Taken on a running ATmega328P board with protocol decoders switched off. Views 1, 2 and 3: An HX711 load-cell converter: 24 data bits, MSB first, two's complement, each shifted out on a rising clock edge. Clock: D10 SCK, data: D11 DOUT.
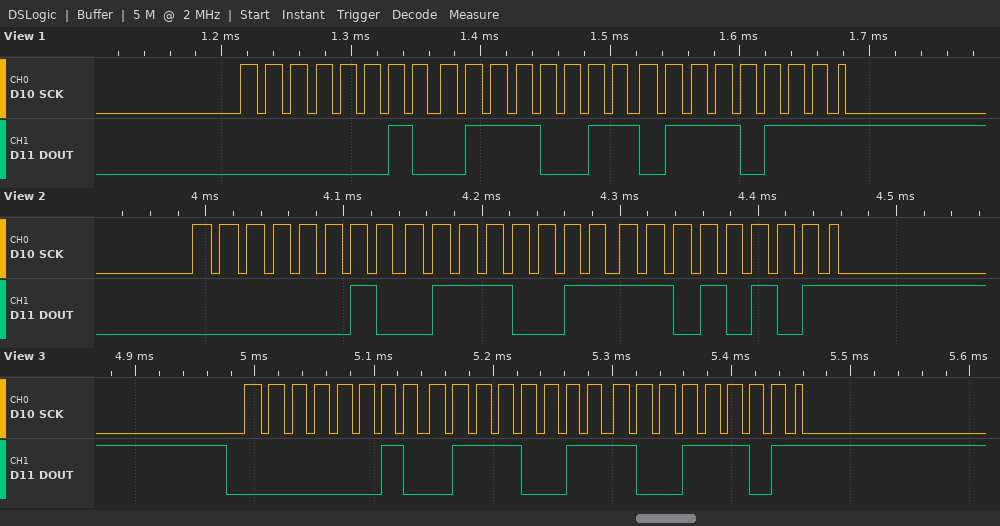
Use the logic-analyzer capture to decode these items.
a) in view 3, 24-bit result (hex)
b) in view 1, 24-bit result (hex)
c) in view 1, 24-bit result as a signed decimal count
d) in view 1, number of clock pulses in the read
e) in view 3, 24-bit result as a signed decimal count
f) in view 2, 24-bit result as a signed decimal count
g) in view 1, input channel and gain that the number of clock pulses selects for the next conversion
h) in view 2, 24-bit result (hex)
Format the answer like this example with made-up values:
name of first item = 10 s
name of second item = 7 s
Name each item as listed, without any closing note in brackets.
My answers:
in view 3, 24-bit result = 0x02739D
in view 1, 24-bit result = 0x027377
in view 1, 24-bit result as a signed decimal count = 160631
in view 1, number of clock pulses in the read = 25
in view 3, 24-bit result as a signed decimal count = 160669
in view 2, 24-bit result as a signed decimal count = 160725
in view 1, input channel and gain that the number of clock pulses selects for the next conversion = channel A, gain 128
in view 2, 24-bit result = 0x0273D5
